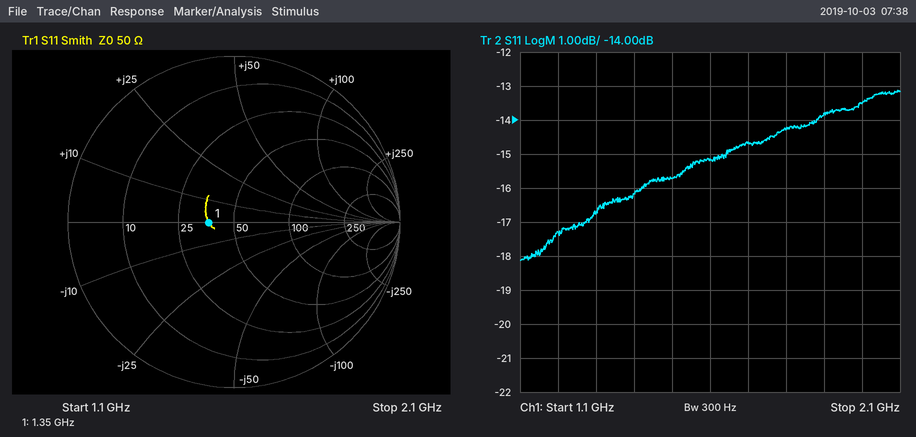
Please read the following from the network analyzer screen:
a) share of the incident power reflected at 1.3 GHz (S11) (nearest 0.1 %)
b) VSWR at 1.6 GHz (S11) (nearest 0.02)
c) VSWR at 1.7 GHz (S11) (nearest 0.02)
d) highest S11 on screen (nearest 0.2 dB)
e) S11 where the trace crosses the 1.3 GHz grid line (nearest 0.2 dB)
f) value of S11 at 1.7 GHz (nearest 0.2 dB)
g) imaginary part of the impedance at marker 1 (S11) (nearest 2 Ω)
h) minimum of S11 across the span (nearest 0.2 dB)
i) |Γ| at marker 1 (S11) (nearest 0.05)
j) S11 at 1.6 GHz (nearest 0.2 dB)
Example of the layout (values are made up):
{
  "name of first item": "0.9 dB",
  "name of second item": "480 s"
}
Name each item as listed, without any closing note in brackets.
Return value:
{
  "share of the incident power reflected at 1.3 GHz (S11)": "2.1 %",
  "VSWR at 1.6 GHz (S11)": "1.42",
  "VSWR at 1.7 GHz (S11)": "1.46",
  "highest S11 on screen": "-13.2 dB",
  "S11 where the trace crosses the 1.3 GHz grid line": "-16.8 dB",
  "value of S11 at 1.7 GHz": "-14.6 dB",
  "imaginary part of the impedance at marker 1 (S11)": "0 Ω",
  "minimum of S11 across the span": "-18.2 dB",
  "|Γ| at marker 1 (S11)": "0.15",
  "S11 at 1.6 GHz": "-15.2 dB"
}
